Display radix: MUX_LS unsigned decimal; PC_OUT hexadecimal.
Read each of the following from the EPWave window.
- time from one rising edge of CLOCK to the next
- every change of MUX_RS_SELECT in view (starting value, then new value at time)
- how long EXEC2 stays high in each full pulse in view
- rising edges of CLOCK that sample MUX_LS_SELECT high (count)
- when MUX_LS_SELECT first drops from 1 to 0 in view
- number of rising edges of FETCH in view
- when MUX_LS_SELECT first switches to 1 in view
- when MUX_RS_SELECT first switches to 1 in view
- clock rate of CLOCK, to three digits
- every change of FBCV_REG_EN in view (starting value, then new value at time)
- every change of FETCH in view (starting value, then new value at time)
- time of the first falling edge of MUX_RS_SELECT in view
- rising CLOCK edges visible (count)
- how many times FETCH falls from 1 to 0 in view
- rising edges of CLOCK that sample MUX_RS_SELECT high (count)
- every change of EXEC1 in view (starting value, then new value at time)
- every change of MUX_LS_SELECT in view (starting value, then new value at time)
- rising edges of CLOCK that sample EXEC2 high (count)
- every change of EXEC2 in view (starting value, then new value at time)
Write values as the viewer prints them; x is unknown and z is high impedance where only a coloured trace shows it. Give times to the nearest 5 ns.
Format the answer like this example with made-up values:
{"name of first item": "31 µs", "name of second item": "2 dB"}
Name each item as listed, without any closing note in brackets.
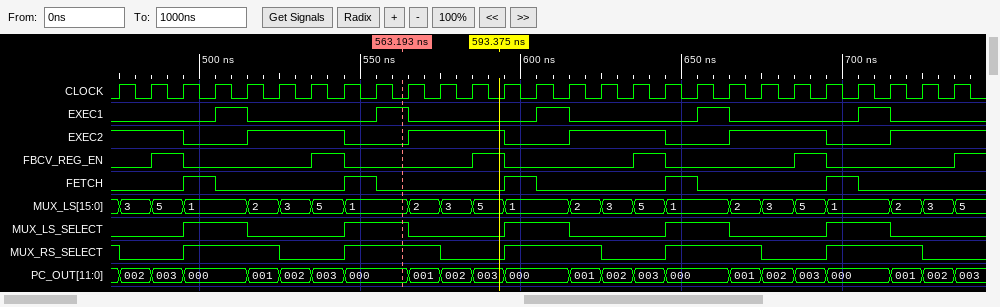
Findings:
{"time from one rising edge of CLOCK to the next": "10 ns", "every change of MUX_RS_SELECT in view": "1, 0 at 475 ns, 1 at 495 ns, 0 at 525 ns, 1 at 545 ns, 0 at 575 ns, 1 at 595 ns, 0 at 625 ns, 1 at 645 ns, 0 at 675 ns, 1 at 695 ns, 0 at 725 ns", "how long EXEC2 stays high in each full pulse in view": "30 ns, 30 ns, 30 ns, 30 ns", "rising edges of CLOCK that sample MUX_LS_SELECT high": "10", "when MUX_LS_SELECT first drops from 1 to 0 in view": "515 ns", "number of rising edges of FETCH in view": "5", "when MUX_LS_SELECT first switches to 1 in view": "495 ns", "when MUX_RS_SELECT first switches to 1 in view": "495 ns", "clock rate of CLOCK, to three digits": "100 MHz", "every change of FBCV_REG_EN in view": "0, 1 at 485 ns, 0 at 495 ns, 1 at 535 ns, 0 at 545 ns, 1 at 585 ns, 0 at 595 ns, 1 at 635 ns, 0 at 645 ns, 1 at 685 ns, 0 at 695 ns, 1 at 735 ns", "every change of FETCH in view": "0, 1 at 495 ns, 0 at 505 ns, 1 at 545 ns, 0 at 555 ns, 1 at 595 ns, 0 at 605 ns, 1 at 645 ns, 0 at 655 ns, 1 at 695 ns, 0 at 705 ns", "time of the first falling edge of MUX_RS_SELECT in view": "475 ns", "rising CLOCK edges visible": "27", "how many times FETCH falls from 1 to 0 in view": "5", "rising edges of CLOCK that sample MUX_RS_SELECT high": "16", "every change of EXEC1 in view": "0, 1 at 505 ns, 0 at 515 ns, 1 at 555 ns, 0 at 565 ns, 1 at 605 ns, 0 at 615 ns, 1 at 655 ns, 0 at 665 ns, 1 at 705 ns, 0 at 715 ns", "every change of MUX_LS_SELECT in view": "0, 1 at 495 ns, 0 at 515 ns, 1 at 545 ns, 0 at 565 ns, 1 at 595 ns, 0 at 615 ns, 1 at 645 ns, 0 at 665 ns, 1 at 695 ns, 0 at 715 ns", "rising edges of CLOCK that sample EXEC2 high": "17", "every change of EXEC2 in view": "1, 0 at 495 ns, 1 at 515 ns, 0 at 545 ns, 1 at 565 ns, 0 at 595 ns, 1 at 615 ns, 0 at 645 ns, 1 at 665 ns, 0 at 695 ns, 1 at 715 ns"}
